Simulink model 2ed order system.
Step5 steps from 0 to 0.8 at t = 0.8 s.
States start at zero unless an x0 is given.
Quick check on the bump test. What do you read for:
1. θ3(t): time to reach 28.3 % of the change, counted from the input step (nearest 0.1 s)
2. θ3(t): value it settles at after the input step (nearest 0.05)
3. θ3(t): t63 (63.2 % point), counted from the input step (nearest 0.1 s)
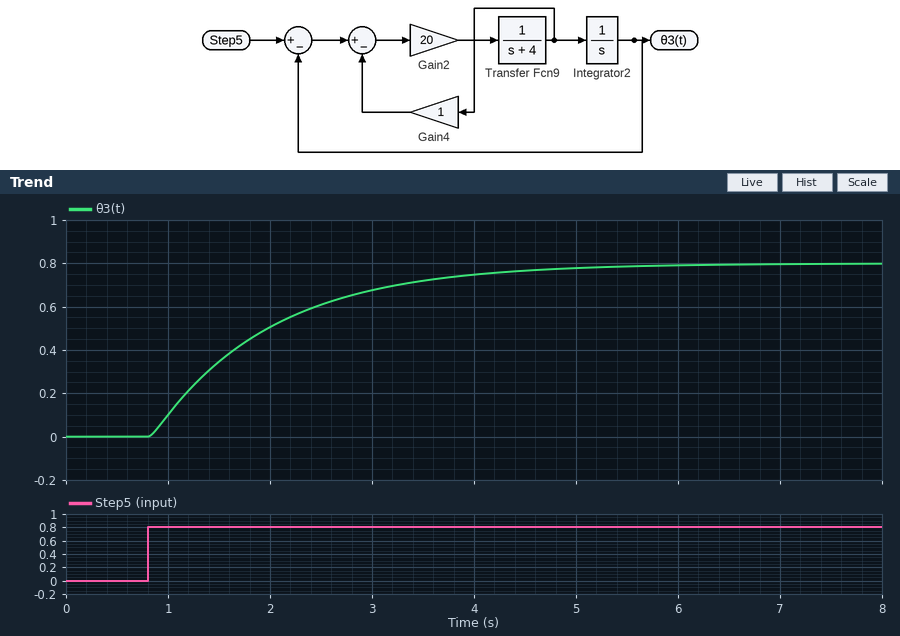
0.4 s
0.80
1.2 s
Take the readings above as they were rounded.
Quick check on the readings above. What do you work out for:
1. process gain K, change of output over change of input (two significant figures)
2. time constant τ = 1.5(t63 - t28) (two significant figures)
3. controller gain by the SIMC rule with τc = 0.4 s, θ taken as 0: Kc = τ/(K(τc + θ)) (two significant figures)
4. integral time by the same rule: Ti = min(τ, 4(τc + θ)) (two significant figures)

1.0
1.2 s
3.0
1.2 s
